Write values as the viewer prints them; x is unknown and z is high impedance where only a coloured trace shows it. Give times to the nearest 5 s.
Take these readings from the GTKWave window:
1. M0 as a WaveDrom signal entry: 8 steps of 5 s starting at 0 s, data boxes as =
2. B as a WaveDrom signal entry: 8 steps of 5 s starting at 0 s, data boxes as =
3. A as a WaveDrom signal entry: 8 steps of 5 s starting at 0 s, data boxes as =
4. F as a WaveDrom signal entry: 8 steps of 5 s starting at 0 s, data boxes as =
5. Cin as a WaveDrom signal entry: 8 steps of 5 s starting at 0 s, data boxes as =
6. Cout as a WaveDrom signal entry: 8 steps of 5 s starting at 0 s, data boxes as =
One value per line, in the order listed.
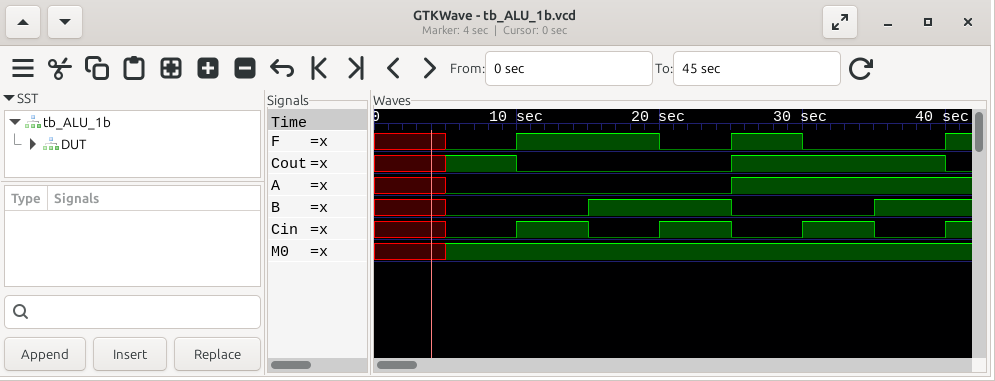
{name: 'M0', wave: 'x1......'}
{name: 'B', wave: 'x0.1.0.1'}
{name: 'A', wave: 'x0...1..'}
{name: 'F', wave: 'x01.010.'}
{name: 'Cin', wave: 'x0101010'}
{name: 'Cout', wave: 'x10..1..'}
